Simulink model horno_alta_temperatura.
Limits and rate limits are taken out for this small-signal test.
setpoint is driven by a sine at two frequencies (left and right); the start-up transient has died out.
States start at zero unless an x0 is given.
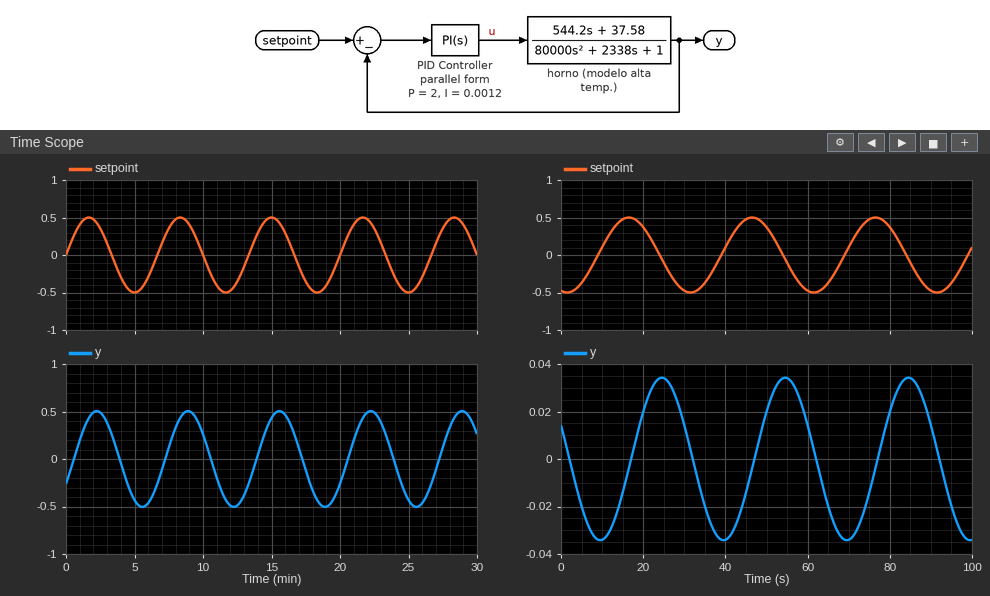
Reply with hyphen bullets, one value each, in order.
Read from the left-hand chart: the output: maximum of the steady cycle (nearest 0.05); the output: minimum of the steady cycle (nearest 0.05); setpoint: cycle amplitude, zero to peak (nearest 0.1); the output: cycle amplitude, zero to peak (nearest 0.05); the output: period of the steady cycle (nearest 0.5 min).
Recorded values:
- 0.50
- -0.50
- 0.5
- 0.50
- 6.5 min
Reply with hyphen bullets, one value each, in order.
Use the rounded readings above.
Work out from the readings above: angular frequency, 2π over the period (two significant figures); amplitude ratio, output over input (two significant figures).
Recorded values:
- 0.97 rad/min
- 1.0
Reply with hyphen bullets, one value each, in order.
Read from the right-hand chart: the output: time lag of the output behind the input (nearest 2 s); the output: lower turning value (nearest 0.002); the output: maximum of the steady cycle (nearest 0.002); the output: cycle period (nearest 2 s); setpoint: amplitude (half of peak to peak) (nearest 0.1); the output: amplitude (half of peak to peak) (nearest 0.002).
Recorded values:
- 8 s
- -0.034
- 0.034
- 30 s
- 0.5
- 0.034
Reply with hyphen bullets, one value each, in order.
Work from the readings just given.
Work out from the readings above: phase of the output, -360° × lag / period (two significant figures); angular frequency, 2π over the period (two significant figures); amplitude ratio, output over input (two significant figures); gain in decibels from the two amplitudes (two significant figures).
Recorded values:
- -96°
- 0.21 rad/s
- 0.068
- -23 dB
